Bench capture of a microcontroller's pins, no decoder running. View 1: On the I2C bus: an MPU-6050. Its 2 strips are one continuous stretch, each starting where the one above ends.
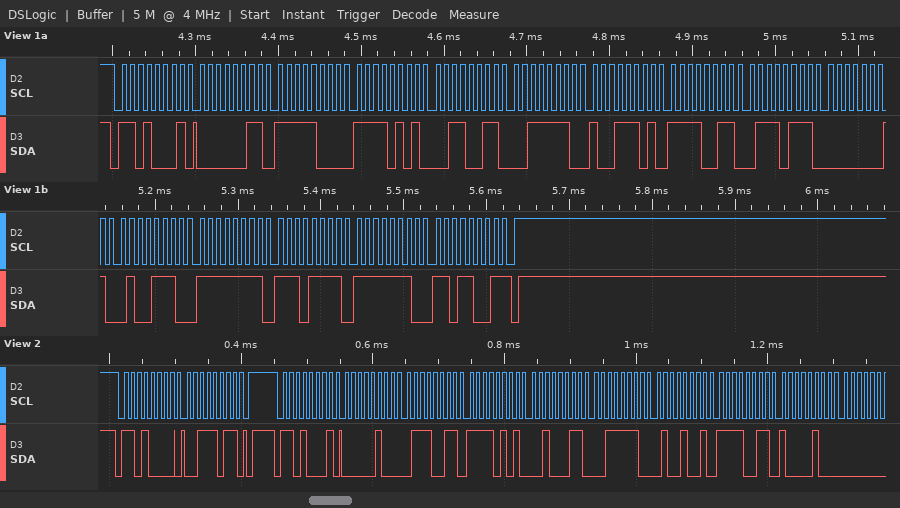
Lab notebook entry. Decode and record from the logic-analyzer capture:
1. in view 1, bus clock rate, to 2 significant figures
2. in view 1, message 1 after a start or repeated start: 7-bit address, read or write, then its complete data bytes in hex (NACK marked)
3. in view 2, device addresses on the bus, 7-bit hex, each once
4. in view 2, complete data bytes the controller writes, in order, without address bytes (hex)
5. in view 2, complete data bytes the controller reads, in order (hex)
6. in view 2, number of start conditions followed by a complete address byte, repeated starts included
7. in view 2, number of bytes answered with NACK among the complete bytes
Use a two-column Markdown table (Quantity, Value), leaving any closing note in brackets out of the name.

| Quantity | Value |
|---|---|
| in view 1, bus clock rate, to 2 significant figures | 100 kHz |
| in view 1, message 1 after a start or repeated start: 7-bit address, read or write, then its complete data bytes in hex | 0x68 read: 03 F8 F5 33 3E 9D F3 77 01 4E FF EF FE D9 NACK |
| in view 2, device addresses on the bus, 7-bit hex, each once | 0x68 |
| in view 2, complete data bytes the controller writes, in order, without address bytes | 3B |
| in view 2, complete data bytes the controller reads, in order | 04 73 F5 23 3E 49 F3 84 |
| in view 2, number of start conditions followed by a complete address byte, repeated starts included | 2 |
| in view 2, number of bytes answered with NACK among the complete bytes | 0 |
